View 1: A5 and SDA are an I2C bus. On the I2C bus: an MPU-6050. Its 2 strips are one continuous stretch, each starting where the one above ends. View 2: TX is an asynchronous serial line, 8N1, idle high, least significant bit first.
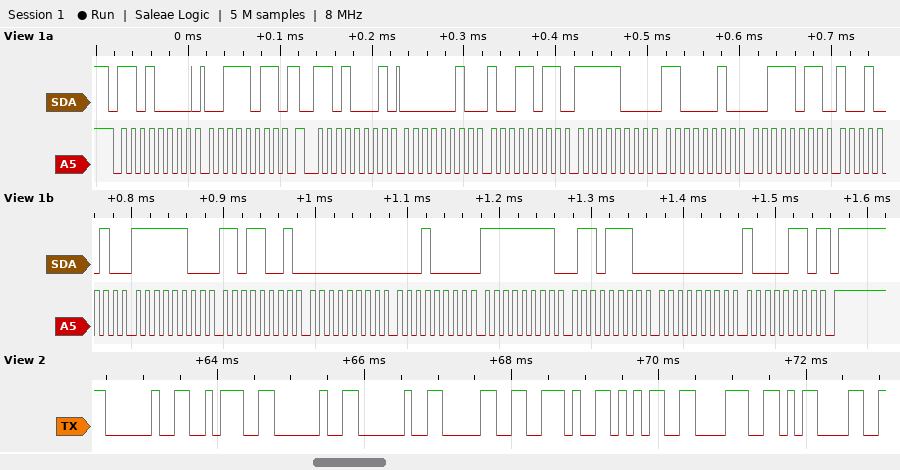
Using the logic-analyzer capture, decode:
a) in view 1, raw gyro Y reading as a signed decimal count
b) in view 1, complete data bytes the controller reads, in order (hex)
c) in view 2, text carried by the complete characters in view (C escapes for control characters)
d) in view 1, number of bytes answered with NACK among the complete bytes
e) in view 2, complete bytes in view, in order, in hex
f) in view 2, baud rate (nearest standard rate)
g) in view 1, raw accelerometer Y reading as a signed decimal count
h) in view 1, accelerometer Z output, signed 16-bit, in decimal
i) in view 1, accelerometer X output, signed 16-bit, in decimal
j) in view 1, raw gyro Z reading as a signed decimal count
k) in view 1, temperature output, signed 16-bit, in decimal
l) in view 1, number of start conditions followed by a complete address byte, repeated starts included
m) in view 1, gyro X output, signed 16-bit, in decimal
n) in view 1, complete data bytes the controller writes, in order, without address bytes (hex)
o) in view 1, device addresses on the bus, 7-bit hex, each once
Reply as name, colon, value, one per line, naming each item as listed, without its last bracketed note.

in view 1, raw gyro Y reading as a signed decimal count: -146
in view 1, complete data bytes the controller reads, in order: 02 9B F8 C2 3B 92 FC D9 00 10 FF 6E 00 86
in view 2, text carried by the complete characters in view: " :  0.58\r"
in view 1, number of bytes answered with NACK among the complete bytes: 1
in view 2, complete bytes in view, in order, in hex: 20 3A 20 20 30 2E 35 38 0D
in view 2, baud rate: 9600 baud
in view 1, raw accelerometer Y reading as a signed decimal count: -1854
in view 1, accelerometer Z output, signed 16-bit, in decimal: 15250
in view 1, accelerometer X output, signed 16-bit, in decimal: 667
in view 1, raw gyro Z reading as a signed decimal count: 134
in view 1, temperature output, signed 16-bit, in decimal: -807
in view 1, number of start conditions followed by a complete address byte, repeated starts included: 2
in view 1, gyro X output, signed 16-bit, in decimal: 16
in view 1, complete data bytes the controller writes, in order, without address bytes: 3B
in view 1, device addresses on the bus, 7-bit hex, each once: 0x68
